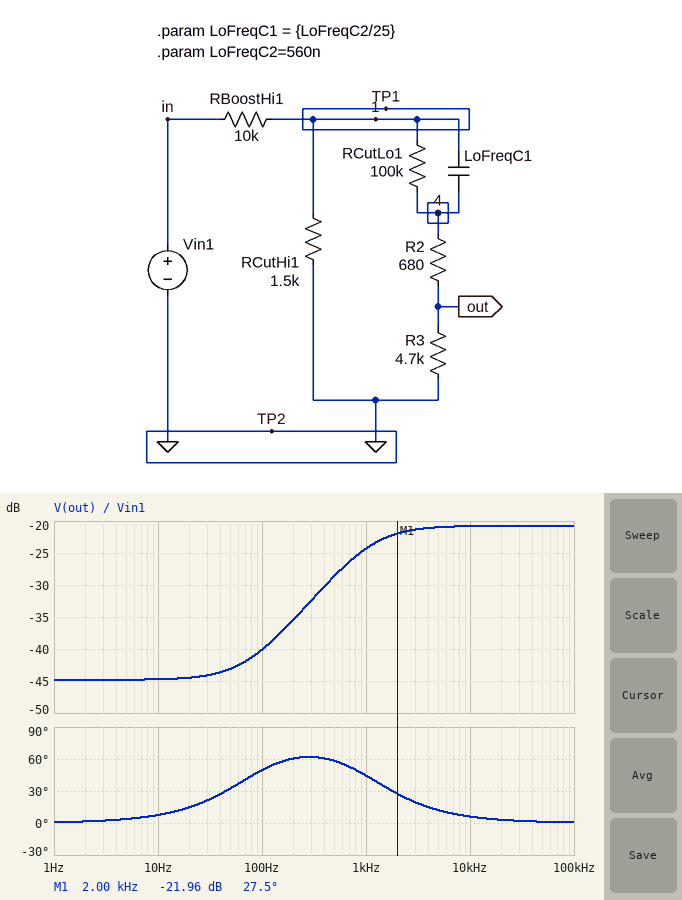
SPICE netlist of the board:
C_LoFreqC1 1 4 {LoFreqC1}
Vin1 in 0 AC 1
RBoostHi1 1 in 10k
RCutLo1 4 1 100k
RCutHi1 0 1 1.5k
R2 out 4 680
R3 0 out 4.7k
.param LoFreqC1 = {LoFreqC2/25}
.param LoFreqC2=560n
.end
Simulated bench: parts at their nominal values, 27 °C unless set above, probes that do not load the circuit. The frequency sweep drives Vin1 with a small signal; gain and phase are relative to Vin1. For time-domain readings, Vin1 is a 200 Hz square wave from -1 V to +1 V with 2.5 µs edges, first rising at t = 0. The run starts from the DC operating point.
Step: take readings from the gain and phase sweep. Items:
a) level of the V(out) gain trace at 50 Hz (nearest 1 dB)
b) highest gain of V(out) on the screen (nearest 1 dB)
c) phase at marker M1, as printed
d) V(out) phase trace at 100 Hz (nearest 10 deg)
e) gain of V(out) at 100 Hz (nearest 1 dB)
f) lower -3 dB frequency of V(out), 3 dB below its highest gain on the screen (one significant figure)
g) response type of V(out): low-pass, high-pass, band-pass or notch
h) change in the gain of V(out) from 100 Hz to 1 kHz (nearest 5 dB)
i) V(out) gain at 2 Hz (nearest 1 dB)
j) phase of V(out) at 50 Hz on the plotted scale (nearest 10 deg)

-43 dB
-21 dB
27.5 deg
50 deg
-40 dB
1 kHz
high-pass
15 dB
-45 dB
30 deg
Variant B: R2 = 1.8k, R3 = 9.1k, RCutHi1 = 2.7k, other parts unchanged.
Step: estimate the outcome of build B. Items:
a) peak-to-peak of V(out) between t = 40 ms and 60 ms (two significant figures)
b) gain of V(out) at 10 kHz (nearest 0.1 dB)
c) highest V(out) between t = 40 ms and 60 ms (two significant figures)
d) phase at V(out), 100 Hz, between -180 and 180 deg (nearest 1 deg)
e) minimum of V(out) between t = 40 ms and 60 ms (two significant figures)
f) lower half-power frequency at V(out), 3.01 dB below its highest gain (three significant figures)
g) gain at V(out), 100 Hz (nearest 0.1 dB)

560 mV
-16.6 dB
280 mV
45 deg
-280 mV
608 Hz
-30.7 dB
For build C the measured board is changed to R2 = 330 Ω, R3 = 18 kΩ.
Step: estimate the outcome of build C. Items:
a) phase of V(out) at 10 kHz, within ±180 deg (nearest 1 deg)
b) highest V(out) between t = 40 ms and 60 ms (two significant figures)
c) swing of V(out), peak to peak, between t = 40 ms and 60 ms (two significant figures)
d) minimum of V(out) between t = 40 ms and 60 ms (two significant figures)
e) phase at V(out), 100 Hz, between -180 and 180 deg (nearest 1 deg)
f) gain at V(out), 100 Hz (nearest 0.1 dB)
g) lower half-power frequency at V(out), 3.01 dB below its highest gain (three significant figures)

2 deg
220 mV
440 mV
-220 mV
42 deg
-29.6 dB
421 Hz
